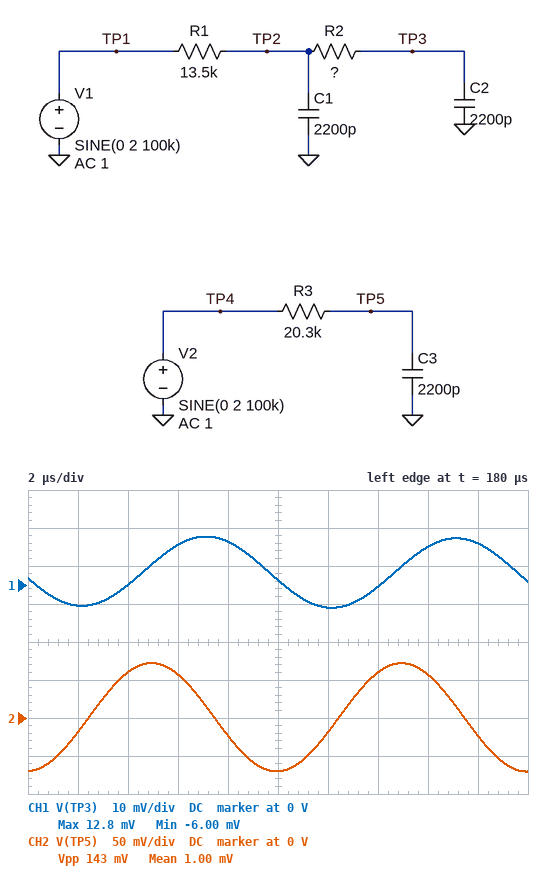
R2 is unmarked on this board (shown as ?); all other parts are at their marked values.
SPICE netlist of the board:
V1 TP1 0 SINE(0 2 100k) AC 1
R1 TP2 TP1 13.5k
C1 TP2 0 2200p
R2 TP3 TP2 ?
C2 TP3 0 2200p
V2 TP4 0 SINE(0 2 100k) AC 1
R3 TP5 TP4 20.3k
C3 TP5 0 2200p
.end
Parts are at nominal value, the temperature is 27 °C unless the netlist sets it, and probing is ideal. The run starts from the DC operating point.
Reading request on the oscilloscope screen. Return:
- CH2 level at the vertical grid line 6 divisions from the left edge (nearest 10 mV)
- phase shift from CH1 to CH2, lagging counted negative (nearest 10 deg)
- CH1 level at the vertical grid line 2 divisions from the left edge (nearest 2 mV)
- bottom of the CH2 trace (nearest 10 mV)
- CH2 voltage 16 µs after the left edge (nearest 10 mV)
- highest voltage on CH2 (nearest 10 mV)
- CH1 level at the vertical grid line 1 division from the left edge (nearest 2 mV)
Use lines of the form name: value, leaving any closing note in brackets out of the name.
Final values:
CH2 level at the vertical grid line 6 divisions from the left edge: -20 mV
phase shift from CH1 to CH2, lagging counted negative: 80 deg
CH1 level at the vertical grid line 2 divisions from the left edge: 0 V
bottom of the CH2 trace: -70 mV
CH2 voltage 16 µs after the left edge: 60 mV
highest voltage on CH2: 70 mV
CH1 level at the vertical grid line 1 division from the left edge: -6 mV
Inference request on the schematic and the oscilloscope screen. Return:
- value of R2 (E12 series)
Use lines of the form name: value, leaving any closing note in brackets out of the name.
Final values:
value of R2: 8.2 kΩ
